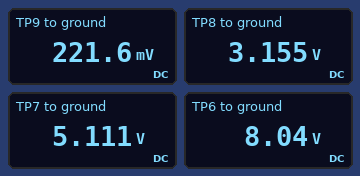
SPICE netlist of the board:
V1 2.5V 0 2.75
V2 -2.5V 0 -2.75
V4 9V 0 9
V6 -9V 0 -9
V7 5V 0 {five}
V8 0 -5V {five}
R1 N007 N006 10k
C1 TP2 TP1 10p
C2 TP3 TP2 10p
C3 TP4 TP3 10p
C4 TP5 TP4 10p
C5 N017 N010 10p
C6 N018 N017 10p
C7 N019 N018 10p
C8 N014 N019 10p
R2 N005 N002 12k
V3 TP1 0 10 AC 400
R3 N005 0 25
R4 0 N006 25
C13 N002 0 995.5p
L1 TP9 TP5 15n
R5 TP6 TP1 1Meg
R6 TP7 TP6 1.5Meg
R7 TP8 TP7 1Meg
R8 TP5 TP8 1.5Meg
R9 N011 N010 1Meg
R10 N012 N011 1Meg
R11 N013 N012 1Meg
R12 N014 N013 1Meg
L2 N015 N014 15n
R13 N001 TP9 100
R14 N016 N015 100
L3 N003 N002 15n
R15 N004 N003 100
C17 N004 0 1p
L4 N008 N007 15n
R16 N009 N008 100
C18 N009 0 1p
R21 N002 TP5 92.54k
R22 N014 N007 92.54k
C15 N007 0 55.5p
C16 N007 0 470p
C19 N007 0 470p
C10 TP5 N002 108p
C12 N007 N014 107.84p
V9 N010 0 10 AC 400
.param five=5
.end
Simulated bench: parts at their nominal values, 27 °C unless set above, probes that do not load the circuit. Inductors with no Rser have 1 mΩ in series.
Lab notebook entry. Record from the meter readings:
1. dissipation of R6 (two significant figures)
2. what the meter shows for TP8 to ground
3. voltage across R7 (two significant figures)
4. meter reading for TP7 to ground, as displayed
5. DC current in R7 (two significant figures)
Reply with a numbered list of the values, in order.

1. 5.7 µW
2. 3.155 V
3. 2.0 V
4. 5.111 V
5. 2.0 µA
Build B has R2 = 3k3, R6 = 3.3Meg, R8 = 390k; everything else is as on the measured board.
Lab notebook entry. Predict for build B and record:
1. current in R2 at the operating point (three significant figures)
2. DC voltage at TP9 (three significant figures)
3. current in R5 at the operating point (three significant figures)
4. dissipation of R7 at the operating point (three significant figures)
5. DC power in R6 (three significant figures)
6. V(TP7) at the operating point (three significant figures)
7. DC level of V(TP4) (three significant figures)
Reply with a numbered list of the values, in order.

1. 2.01 µA
2. 191 mV
3. 1.72 µA
4. 2.97 µW
5. 9.81 µW
6. 2.59 V
7. 2.64 V
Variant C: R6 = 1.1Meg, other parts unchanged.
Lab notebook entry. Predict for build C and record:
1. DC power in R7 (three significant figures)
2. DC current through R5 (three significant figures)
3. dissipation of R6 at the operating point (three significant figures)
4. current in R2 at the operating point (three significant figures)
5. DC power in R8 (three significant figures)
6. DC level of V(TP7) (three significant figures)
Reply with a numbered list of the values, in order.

1. 4.51 µW
2. 2.12 µA
3. 4.96 µW
4. 2.09 µA
5. 6.76 µW
6. 5.54 V
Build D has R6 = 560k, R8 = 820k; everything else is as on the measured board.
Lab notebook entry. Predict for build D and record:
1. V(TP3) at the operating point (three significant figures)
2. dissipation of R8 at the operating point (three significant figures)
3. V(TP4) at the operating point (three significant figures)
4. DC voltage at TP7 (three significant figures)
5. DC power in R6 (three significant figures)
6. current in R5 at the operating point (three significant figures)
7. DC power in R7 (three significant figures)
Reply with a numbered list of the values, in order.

1. 5.14 V
2. 6.78 µW
3. 2.71 V
4. 5.51 V
5. 4.63 µW
6. 2.88 µA
7. 8.27 µW
